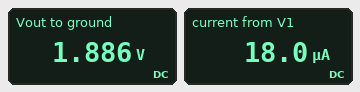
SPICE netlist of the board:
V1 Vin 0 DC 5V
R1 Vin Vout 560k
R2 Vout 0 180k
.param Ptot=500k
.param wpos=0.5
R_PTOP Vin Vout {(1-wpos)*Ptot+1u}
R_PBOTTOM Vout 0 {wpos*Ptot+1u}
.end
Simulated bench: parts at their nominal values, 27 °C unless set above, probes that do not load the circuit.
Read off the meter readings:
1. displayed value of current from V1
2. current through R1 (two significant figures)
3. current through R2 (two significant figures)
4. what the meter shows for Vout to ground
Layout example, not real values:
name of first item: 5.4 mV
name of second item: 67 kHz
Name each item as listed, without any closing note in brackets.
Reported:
displayed value of current from V1: 18.0 µA
current through R1: 5.6 µA
current through R2: 10 µA
what the meter shows for Vout to ground: 1.886 V
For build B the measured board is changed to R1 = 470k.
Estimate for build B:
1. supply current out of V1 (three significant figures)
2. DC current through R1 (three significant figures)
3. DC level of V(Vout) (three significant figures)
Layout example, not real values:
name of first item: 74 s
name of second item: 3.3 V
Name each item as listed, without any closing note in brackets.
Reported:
supply current out of V1: 18.7 µA
DC current through R1: 6.48 µA
DC level of V(Vout): 1.95 V
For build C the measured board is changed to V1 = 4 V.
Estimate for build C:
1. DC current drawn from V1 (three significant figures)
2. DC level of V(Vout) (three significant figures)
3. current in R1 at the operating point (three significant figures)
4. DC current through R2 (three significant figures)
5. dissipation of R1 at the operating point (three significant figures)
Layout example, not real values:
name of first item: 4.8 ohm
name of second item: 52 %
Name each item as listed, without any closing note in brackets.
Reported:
DC current drawn from V1: 14.4 µA
DC level of V(Vout): 1.51 V
current in R1 at the operating point: 4.45 µA
DC current through R2: 8.38 µA
dissipation of R1 at the operating point: 11.1 µW
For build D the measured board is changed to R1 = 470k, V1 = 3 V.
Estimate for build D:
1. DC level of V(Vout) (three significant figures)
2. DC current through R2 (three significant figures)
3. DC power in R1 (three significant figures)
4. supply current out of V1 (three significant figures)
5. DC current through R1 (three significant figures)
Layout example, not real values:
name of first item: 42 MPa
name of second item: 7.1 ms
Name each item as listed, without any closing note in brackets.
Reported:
DC level of V(Vout): 1.17 V
DC current through R2: 6.51 µA
DC power in R1: 7.11 µW
supply current out of V1: 11.2 µA
DC current through R1: 3.89 µA
